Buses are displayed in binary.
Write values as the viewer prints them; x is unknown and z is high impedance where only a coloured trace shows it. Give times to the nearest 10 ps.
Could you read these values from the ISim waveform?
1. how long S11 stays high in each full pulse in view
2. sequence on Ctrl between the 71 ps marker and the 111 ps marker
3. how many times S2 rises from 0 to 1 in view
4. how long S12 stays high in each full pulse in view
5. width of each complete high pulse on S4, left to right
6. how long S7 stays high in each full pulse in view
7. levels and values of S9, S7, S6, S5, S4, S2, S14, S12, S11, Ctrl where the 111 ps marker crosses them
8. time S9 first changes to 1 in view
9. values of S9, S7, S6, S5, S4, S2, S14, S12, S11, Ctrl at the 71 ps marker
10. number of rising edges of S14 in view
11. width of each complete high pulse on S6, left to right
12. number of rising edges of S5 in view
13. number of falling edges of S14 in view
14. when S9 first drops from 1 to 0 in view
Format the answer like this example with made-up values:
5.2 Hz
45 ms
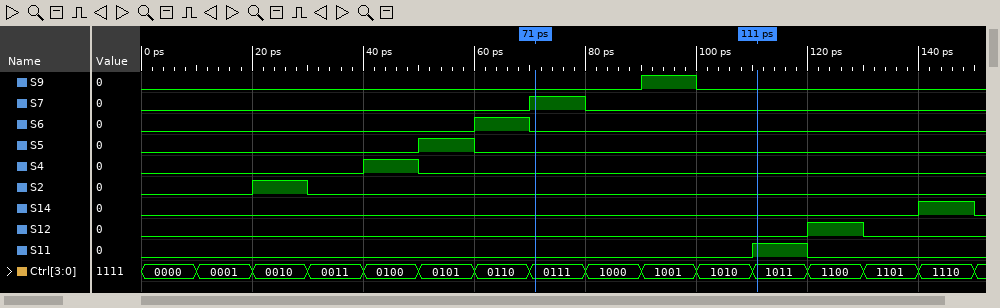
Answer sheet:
10 ps
0111, 1000, 1001, 1010, 1011
1
10 ps
10 ps
10 ps
S9=0, S7=0, S6=0, S5=0, S4=0, S2=0, S14=0, S12=0, S11=1, Ctrl=1011
90 ps
S9=0, S7=1, S6=0, S5=0, S4=0, S2=0, S14=0, S12=0, S11=0, Ctrl=0111
1
10 ps
1
1
100 ps
